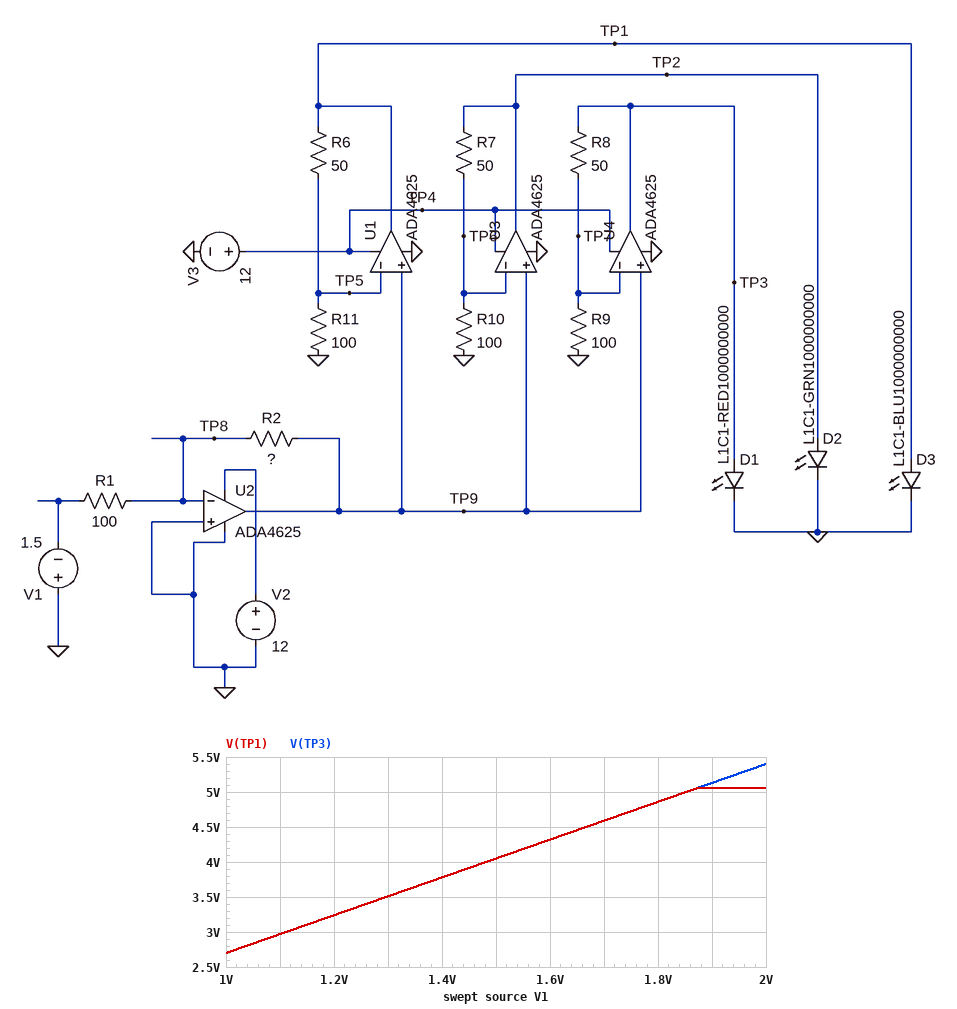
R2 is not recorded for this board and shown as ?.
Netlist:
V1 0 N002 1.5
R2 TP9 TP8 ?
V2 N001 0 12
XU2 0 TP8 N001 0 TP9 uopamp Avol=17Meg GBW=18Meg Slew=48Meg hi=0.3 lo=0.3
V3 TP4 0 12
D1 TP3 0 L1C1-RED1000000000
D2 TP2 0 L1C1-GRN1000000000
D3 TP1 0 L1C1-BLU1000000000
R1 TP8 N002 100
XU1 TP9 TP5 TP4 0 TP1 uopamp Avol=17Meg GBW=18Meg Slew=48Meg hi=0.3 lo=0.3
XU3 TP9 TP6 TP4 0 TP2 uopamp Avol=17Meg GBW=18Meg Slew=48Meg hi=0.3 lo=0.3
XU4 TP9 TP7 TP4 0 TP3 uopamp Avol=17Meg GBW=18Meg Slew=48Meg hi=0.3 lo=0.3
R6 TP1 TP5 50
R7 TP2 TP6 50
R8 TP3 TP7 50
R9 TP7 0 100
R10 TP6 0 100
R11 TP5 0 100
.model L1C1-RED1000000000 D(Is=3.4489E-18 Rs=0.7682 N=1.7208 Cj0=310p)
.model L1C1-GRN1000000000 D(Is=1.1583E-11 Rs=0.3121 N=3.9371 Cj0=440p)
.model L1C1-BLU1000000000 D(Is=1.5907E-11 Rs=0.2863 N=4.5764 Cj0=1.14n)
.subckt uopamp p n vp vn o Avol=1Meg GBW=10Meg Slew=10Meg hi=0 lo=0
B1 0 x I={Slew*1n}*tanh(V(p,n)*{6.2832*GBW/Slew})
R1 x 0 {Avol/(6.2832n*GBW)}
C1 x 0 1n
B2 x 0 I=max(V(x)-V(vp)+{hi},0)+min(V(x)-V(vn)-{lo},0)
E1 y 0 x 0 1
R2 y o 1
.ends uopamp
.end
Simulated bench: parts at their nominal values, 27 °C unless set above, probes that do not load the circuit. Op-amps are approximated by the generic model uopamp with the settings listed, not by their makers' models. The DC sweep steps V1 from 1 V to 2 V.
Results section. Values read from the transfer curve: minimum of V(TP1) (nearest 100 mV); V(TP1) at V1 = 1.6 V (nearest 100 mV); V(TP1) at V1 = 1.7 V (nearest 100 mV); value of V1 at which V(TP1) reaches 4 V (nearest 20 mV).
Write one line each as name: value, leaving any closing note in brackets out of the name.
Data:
minimum of V(TP1): 2.7 V
V(TP1) at V1 = 1.6 V: 4.3 V
V(TP1) at V1 = 1.7 V: 4.6 V
value of V1 at which V(TP1) reaches 4 V: 1.48 V
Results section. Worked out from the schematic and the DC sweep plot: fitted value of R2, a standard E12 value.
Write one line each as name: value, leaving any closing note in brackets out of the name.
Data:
fitted value of R2, a standard E12 value: 180 Ω
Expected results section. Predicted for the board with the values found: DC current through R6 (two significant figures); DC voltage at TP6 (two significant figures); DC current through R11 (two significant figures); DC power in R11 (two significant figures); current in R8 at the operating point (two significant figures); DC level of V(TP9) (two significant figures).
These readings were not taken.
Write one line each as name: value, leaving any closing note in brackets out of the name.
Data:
DC current through R6: 27 mA
DC voltage at TP6: 2.7 V
DC current through R11: 27 mA
DC power in R11: 73 mW
current in R8 at the operating point: 27 mA
DC level of V(TP9): 2.7 V
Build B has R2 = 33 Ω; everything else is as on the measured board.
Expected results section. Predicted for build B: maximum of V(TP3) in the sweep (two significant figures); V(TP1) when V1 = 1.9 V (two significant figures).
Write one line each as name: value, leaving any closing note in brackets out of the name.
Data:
maximum of V(TP3) in the sweep: 990 mV
V(TP1) when V1 = 1.9 V: 940 mV
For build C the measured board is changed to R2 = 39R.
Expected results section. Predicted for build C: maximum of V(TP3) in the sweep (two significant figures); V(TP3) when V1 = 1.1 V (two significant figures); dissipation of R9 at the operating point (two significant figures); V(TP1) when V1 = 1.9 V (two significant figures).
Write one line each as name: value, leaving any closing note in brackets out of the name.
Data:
maximum of V(TP3) in the sweep: 1.2 V
V(TP3) when V1 = 1.1 V: 640 mV
dissipation of R9 at the operating point: 3.4 mW
V(TP1) when V1 = 1.9 V: 1.1 V
